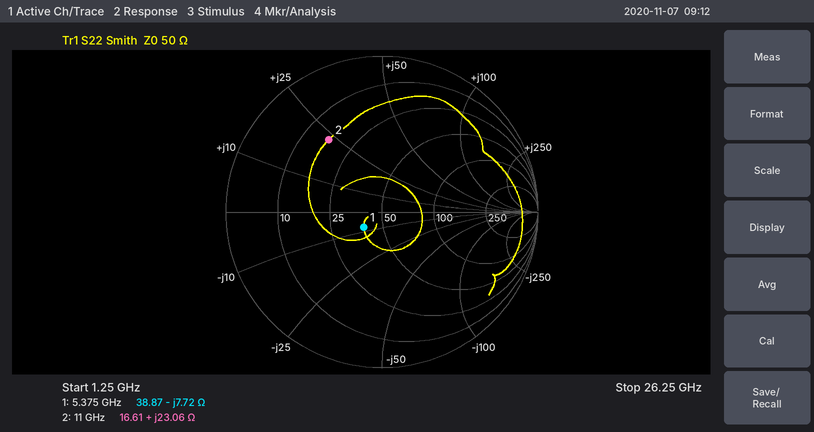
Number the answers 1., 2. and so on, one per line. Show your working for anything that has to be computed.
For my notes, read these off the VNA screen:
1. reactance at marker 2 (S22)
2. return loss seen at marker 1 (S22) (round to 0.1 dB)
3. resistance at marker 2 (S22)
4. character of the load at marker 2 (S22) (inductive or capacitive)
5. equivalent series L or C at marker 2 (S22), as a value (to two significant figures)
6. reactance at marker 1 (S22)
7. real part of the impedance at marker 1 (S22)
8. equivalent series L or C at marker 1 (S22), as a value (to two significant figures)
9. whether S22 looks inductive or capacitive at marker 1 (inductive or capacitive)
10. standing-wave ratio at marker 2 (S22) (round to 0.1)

1. +23.06 Ω
2. 16.4 dB
3. 16.61 Ω
4. inductive
5. L = 23.06 Ω/(2π × 11 GHz) ≈ 334 pH, so 330 pH to two significant figures
6. -7.72 Ω
7. 38.87 Ω
8. C = 1/(2π × 5.375 GHz × 7.72 Ω) ≈ 3.8 pF
9. capacitive
10. 3.7
